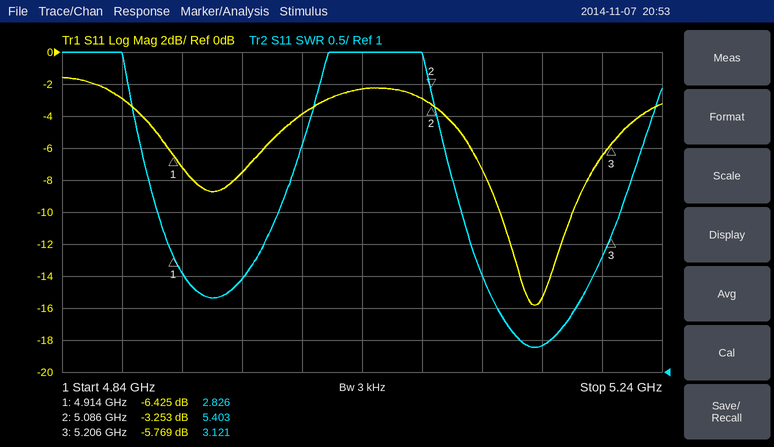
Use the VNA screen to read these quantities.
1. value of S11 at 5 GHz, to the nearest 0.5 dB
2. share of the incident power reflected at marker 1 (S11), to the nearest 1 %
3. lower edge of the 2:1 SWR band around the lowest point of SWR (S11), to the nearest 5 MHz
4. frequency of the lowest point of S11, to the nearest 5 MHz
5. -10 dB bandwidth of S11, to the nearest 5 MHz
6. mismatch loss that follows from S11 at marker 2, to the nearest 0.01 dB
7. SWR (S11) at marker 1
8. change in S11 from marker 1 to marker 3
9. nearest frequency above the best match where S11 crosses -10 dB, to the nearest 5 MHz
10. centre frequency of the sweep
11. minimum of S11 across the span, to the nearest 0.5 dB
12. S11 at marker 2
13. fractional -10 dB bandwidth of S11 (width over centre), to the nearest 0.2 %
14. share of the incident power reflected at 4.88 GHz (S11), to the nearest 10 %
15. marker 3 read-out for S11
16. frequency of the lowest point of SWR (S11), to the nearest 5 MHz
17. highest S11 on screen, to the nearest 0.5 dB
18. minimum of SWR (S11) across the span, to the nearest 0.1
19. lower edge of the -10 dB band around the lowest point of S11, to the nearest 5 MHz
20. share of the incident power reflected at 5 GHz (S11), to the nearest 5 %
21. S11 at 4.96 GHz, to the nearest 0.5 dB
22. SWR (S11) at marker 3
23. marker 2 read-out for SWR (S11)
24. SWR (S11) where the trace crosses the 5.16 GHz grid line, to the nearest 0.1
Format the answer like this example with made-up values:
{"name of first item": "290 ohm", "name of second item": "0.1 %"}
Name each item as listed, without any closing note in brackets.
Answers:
{"value of S11 at 5 GHz, to the nearest 0.5 dB": "-4.0 dB", "share of the incident power reflected at marker 1 (S11), to the nearest 1 %": "23 %", "lower edge of the 2:1 SWR band around the lowest point of SWR (S11), to the nearest 5 MHz": "5.130 GHz", "frequency of the lowest point of S11, to the nearest 5 MHz": "5.155 GHz", "-10 dB bandwidth of S11, to the nearest 5 MHz": "50 MHz", "mismatch loss that follows from S11 at marker 2, to the nearest 0.01 dB": "2.78 dB", "SWR (S11) at marker 1": "2.826", "change in S11 from marker 1 to marker 3": "0.656 dB", "nearest frequency above the best match where S11 crosses -10 dB, to the nearest 5 MHz": "5.180 GHz", "centre frequency of the sweep": "5.04 GHz", "minimum of S11 across the span, to the nearest 0.5 dB": "-16.0 dB", "S11 at marker 2": "-3.253 dB", "fractional -10 dB bandwidth of S11 (width over centre), to the nearest 0.2 %": "1.0 %", "share of the incident power reflected at 4.88 GHz (S11), to the nearest 10 %": "50 %", "marker 3 read-out for S11": "-5.769 dB", "frequency of the lowest point of SWR (S11), to the nearest 5 MHz": "5.155 GHz", "highest S11 on screen, to the nearest 0.5 dB": "-1.5 dB", "minimum of SWR (S11) across the span, to the nearest 0.1": "1.4", "lower edge of the -10 dB band around the lowest point of S11, to the nearest 5 MHz": "5.130 GHz", "share of the incident power reflected at 5 GHz (S11), to the nearest 5 %": "40 %", "S11 at 4.96 GHz, to the nearest 0.5 dB": "-7.5 dB", "SWR (S11) at marker 3": "3.121", "marker 2 read-out for SWR": "5.403", "SWR (S11) where the trace crosses the 5.16 GHz grid line, to the nearest 0.1": "1.4"}
